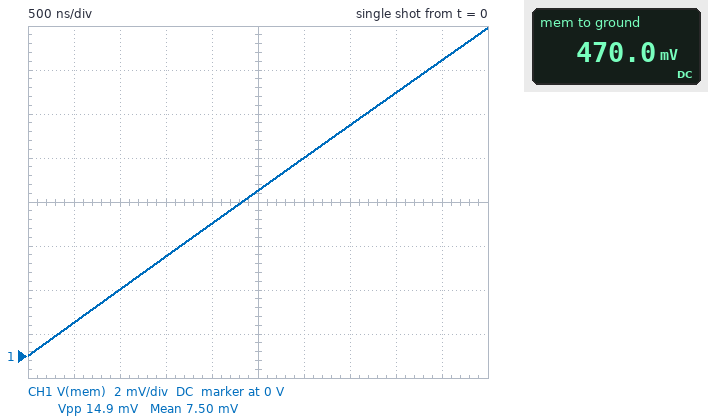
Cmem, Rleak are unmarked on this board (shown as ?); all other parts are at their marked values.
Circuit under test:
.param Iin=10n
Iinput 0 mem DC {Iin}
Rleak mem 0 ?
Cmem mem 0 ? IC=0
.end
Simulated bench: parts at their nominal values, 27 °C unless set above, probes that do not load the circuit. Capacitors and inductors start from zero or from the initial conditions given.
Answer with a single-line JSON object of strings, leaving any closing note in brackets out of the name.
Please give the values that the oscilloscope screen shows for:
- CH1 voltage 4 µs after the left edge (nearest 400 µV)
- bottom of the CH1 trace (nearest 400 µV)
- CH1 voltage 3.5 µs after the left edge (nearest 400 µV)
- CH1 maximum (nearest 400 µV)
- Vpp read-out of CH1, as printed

{"CH1 voltage 4 µs after the left edge": "12.0 mV", "bottom of the CH1 trace": "0 V", "CH1 voltage 3.5 µs after the left edge": "10.4 mV", "CH1 maximum": "14.8 mV", "Vpp read-out of CH1, as printed": "14.9 mV"}
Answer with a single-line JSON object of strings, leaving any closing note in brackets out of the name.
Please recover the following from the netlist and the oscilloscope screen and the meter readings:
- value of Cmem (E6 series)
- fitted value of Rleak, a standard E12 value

{"value of Cmem": "3.3 pF", "fitted value of Rleak, a standard E12 value": "47 MΩ"}
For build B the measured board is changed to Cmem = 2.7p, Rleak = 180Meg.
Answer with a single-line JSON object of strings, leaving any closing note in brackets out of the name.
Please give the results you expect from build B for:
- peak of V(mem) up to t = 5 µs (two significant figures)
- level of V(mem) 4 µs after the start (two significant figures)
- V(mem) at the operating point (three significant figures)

{"peak of V(mem) up to t = 5 µs": "18 mV", "level of V(mem) 4 µs after the start": "15 mV", "V(mem) at the operating point": "1.80 V"}
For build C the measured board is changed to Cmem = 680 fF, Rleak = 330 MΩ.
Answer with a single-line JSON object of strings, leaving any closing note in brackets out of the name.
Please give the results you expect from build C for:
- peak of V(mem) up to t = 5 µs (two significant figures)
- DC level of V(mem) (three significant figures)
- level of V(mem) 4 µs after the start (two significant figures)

{"peak of V(mem) up to t = 5 µs": "73 mV", "DC level of V(mem)": "3.30 V", "level of V(mem) 4 µs after the start": "58 mV"}
